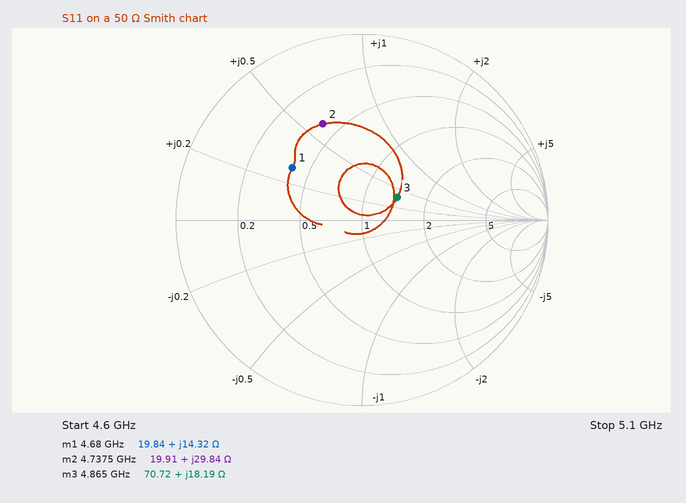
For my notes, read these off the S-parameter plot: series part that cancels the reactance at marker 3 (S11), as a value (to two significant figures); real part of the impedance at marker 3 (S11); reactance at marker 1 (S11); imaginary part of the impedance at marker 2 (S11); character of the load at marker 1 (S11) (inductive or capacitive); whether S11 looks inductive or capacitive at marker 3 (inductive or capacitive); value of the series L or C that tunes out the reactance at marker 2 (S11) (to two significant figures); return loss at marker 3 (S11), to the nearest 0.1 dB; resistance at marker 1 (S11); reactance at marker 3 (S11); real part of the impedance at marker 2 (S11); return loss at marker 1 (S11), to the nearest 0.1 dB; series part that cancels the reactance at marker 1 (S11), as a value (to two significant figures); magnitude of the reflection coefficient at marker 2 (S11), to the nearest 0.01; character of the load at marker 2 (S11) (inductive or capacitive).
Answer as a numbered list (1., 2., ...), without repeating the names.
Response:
1. 1.8 pF
2. 70.72 Ω
3. +14.32 Ω
4. +29.84 Ω
5. inductive
6. inductive
7. 1.1 pF
8. 12.9 dB
9. 19.84 Ω
10. +18.19 Ω
11. 19.91 Ω
12. 6.6 dB
13. 2.4 pF
14. 0.56
15. inductive
